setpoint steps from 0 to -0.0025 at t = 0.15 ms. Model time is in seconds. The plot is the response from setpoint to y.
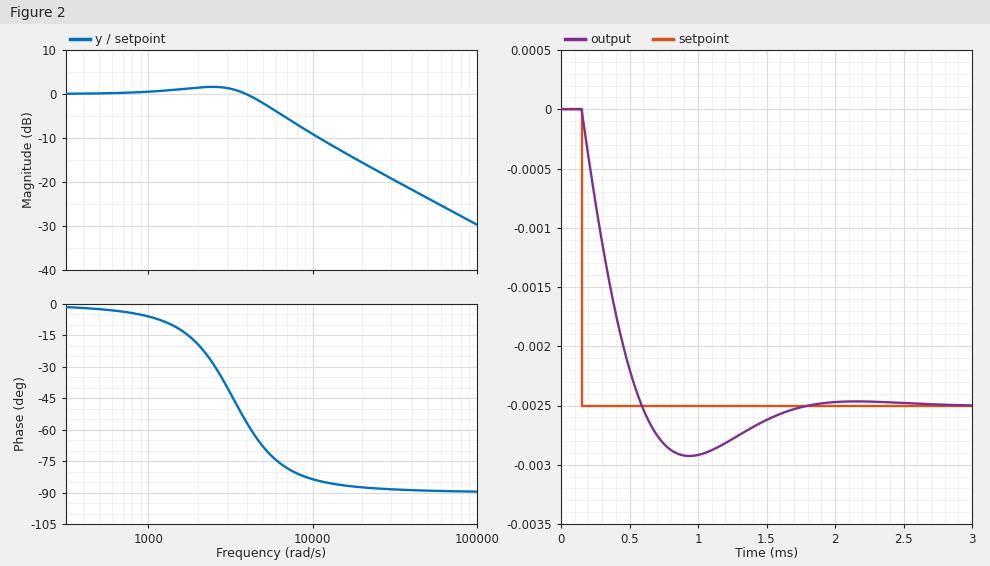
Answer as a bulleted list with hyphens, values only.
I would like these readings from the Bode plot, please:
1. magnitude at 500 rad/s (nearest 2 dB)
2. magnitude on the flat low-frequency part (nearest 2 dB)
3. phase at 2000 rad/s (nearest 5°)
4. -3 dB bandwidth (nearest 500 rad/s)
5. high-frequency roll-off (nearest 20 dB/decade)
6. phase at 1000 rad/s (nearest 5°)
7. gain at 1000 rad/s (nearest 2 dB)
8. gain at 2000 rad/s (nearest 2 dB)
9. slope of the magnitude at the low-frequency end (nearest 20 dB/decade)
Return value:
- 0 dB
- 0 dB
- -20°
- 5500 rad/s
- -20 dB/decade
- -5°
- 0 dB
- 2 dB
- 0 dB/decade
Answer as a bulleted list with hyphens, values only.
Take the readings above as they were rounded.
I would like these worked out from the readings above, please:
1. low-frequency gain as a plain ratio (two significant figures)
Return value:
- 1.0
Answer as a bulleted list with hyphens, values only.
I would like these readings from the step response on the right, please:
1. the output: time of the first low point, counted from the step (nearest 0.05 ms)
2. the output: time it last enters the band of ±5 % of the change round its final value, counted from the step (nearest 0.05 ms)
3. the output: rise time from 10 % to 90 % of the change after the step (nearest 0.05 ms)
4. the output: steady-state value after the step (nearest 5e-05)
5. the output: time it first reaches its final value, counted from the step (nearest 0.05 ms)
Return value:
- 0.80 ms
- 1.35 ms
- 0.35 ms
- -0.00250
- 0.45 ms
